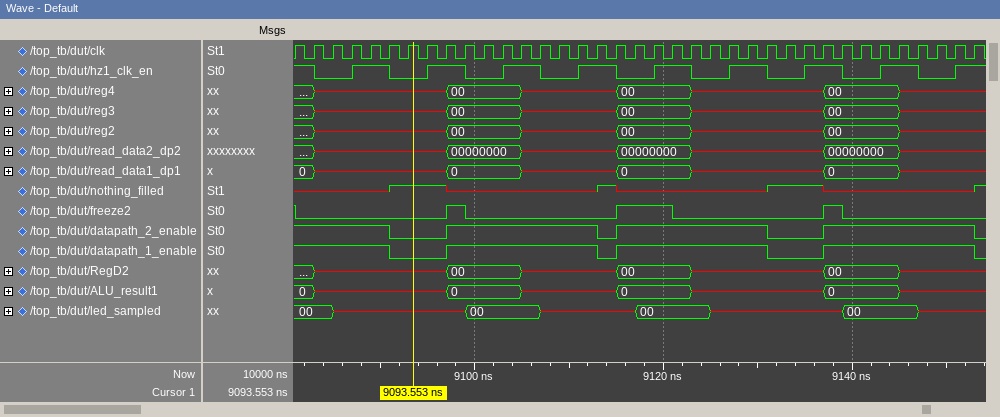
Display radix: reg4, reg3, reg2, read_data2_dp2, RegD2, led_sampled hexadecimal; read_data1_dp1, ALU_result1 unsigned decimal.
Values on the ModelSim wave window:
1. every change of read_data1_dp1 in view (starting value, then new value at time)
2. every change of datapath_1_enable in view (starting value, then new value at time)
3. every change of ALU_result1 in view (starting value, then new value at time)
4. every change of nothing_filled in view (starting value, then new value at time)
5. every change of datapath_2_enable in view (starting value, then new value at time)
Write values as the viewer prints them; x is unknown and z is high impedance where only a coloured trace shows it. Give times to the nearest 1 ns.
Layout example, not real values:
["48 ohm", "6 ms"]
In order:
["0, x at 9083 ns, 0 at 9097 ns, x at 9105 ns, 0 at 9115 ns, x at 9123 ns, 0 at 9137 ns, x at 9145 ns", "1, 0 at 9091 ns, 1 at 9097 ns, 0 at 9113 ns, 1 at 9115 ns, 0 at 9131 ns, 1 at 9137 ns, 0 at 9153 ns", "0, x at 9083 ns, 0 at 9097 ns, x at 9105 ns, 0 at 9115 ns, x at 9123 ns, 0 at 9137 ns, x at 9145 ns", "x, 1 at 9091 ns, x at 9097 ns, 1 at 9113 ns, x at 9115 ns, 1 at 9131 ns, x at 9137 ns, 1 at 9153 ns", "1, 0 at 9091 ns, 1 at 9097 ns, 0 at 9113 ns, 1 at 9115 ns, 0 at 9131 ns, 1 at 9137 ns, 0 at 9153 ns"]
